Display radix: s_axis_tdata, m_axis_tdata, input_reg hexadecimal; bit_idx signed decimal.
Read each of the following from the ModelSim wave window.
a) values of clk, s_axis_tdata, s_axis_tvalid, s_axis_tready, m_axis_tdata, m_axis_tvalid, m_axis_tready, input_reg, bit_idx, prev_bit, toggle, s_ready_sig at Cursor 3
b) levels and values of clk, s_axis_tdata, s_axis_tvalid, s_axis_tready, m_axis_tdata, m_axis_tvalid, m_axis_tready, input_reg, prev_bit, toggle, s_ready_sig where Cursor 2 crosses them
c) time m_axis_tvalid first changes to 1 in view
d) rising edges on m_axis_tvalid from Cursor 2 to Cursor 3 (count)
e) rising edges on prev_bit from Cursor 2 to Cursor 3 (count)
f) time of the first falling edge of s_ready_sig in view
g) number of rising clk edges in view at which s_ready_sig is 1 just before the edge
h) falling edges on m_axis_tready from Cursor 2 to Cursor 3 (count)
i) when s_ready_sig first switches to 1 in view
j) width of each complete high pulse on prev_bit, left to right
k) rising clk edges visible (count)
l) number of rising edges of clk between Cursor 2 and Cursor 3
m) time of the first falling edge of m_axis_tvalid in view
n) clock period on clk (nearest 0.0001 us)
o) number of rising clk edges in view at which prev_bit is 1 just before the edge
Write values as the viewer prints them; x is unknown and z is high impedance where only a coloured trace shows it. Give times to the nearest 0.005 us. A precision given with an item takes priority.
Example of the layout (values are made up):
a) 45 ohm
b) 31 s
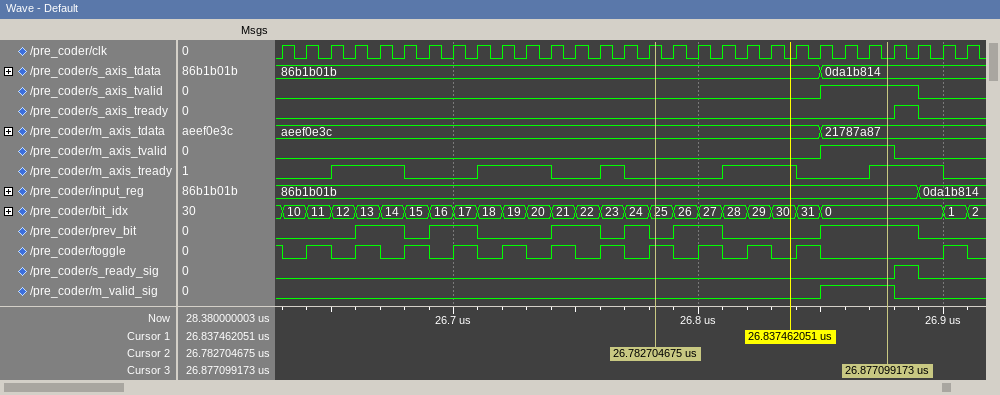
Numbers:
a) clk=0, s_axis_tdata=0da1b814, s_axis_tvalid=1, s_axis_tready=0, m_axis_tdata=21787a87, m_axis_tvalid=1, m_axis_tready=1, input_reg=86b1b01b, bit_idx=0, prev_bit=1, toggle=0, s_ready_sig=0
b) clk=1, s_axis_tdata=86b1b01b, s_axis_tvalid=0, s_axis_tready=0, m_axis_tdata=aeef0e3c, m_axis_tvalid=0, m_axis_tready=0, input_reg=86b1b01b, prev_bit=0, toggle=1, s_ready_sig=0
c) 26.85 us
d) 1
e) 2
f) 26.89 us
g) 1
h) 1
i) 26.88 us
j) 0.02 us, 0.02 us, 0.02 us, 0.01 us, 0.02 us, 0.04 us
k) 29
l) 9
m) 26.88 us
n) 0.01 us
o) 13
